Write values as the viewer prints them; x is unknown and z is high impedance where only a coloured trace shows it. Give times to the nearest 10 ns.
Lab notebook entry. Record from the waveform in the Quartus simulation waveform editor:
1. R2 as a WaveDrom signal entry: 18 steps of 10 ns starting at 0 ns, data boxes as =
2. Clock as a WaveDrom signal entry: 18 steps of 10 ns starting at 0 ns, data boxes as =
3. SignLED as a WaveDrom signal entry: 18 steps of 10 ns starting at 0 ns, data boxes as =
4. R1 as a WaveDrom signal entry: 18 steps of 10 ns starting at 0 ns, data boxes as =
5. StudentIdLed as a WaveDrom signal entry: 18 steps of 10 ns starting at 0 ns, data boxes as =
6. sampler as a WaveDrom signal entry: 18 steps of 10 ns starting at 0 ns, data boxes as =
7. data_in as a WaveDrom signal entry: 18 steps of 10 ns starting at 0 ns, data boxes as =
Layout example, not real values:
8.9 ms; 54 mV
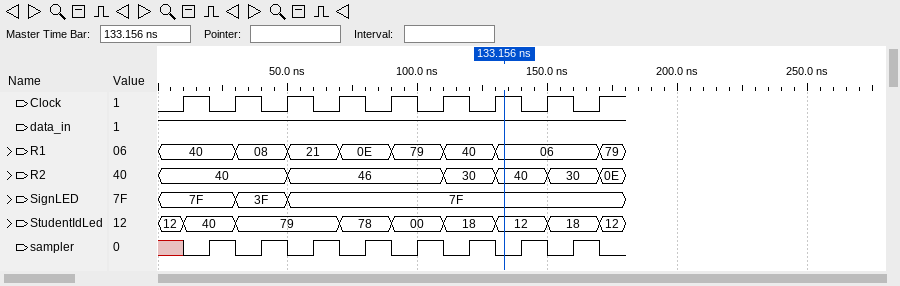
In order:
{name: 'R2', wave: '=....=.....=.=.=.=', data: '40 46 30 40 30 0E'}; {name: 'Clock', wave: '010101010101010101'}; {name: 'SignLED', wave: '=..=.=............', data: '7F 3F 7F'}; {name: 'R1', wave: '=..=.=.=.=.=.=...=', data: '40 08 21 0E 79 40 06 79'}; {name: 'StudentIdLed', wave: '==.=...=.=.=.=.=.=', data: '12 40 79 78 00 18 12 18 12'}; {name: 'sampler', wave: 'x01010101010101010'}; {name: 'data_in', wave: '1.................'}
